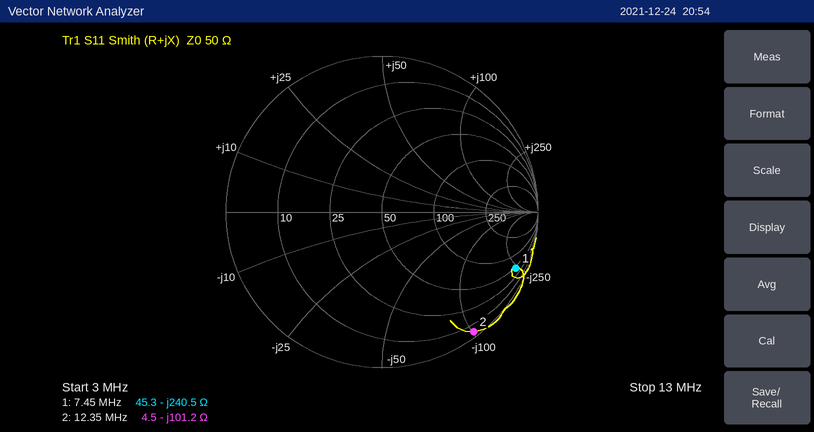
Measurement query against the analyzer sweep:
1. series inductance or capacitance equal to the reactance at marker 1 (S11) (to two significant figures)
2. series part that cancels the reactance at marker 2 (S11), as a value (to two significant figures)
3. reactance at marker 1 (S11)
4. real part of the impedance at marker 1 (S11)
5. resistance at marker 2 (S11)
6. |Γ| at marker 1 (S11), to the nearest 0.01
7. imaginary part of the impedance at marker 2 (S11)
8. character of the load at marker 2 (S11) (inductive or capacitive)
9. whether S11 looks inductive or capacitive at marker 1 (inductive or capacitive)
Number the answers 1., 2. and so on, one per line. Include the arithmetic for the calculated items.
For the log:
1. C = 1/(2π × 7.45 MHz × 240.5 Ω) ≈ 89 pF
2. L = 101.2 Ω/(2π × 12.35 MHz) ≈ 1.3 µH
3. -240.5 Ω
4. 45.3 Ω
5. 4.5 Ω
6. 0.93
7. -101.2 Ω
8. capacitive
9. capacitive
